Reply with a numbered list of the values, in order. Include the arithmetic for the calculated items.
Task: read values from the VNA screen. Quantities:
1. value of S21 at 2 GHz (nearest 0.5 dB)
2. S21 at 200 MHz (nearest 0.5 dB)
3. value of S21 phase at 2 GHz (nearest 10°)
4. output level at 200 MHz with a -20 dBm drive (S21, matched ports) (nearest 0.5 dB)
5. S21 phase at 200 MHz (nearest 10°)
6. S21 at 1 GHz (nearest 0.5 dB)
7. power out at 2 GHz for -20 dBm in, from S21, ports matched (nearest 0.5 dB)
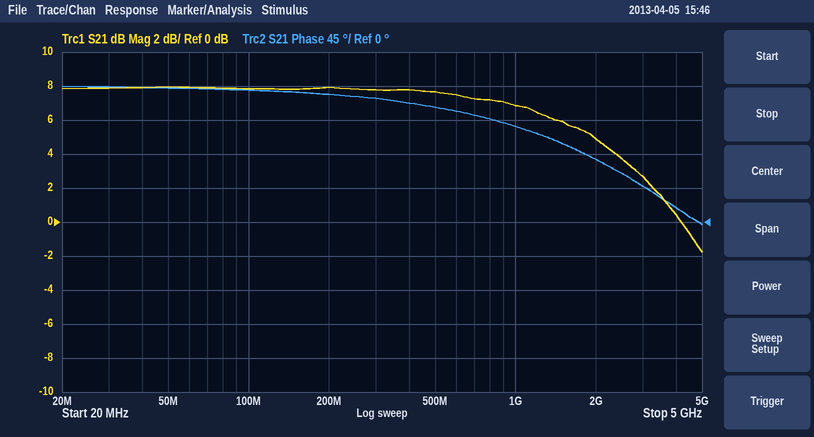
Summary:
1. 5.0 dB
2. 8.0 dB
3. 80°
4. -20 dBm + (8.0 dB) = -12.0 dBm
5. 170°
6. 7.0 dB
7. -20 dBm + (5.0 dB) = -15.0 dBm
